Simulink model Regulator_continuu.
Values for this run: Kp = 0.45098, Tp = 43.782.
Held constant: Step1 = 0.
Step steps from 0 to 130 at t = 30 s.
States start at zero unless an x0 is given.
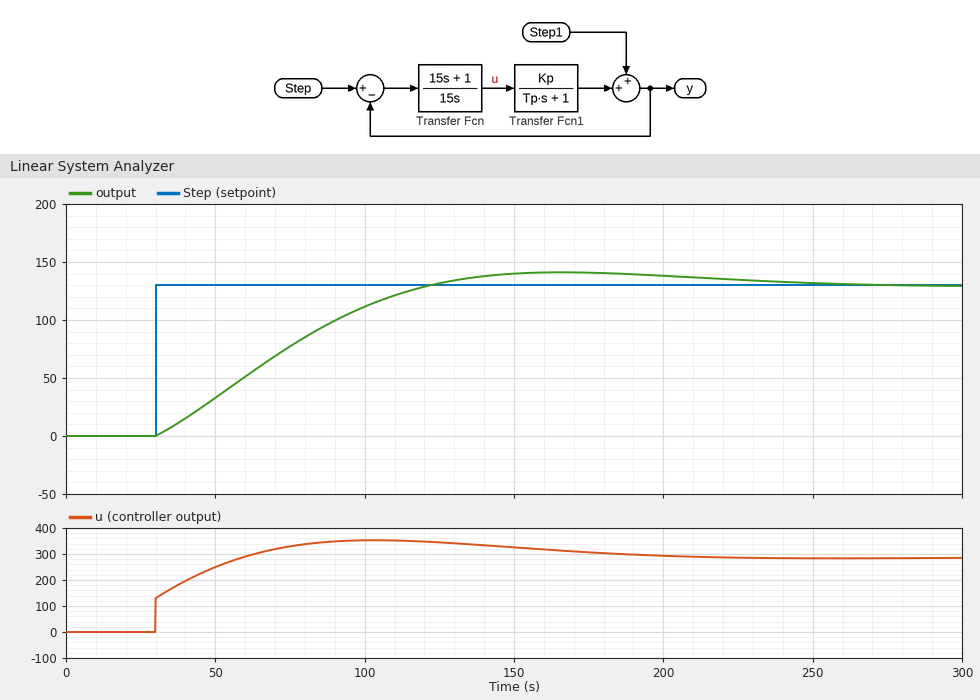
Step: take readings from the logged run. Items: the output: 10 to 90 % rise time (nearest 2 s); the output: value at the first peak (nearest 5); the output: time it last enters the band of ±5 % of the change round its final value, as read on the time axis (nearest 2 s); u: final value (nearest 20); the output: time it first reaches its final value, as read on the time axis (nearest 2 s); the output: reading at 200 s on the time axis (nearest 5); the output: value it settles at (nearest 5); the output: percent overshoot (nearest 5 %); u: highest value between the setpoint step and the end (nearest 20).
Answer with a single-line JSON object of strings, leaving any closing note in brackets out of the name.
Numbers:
{"the output: 10 to 90 % rise time": "66 s", "the output: value at the first peak": "140", "the output: time it last enters the band of ±5 % of the change round its final value, as read on the time axis": "212 s", "u: final value": "280", "the output: time it first reaches its final value, as read on the time axis": "122 s", "the output: reading at 200 s on the time axis": "140", "the output: value it settles at": "130", "the output: percent overshoot": "10 %", "u: highest value between the setpoint step and the end": "360"}
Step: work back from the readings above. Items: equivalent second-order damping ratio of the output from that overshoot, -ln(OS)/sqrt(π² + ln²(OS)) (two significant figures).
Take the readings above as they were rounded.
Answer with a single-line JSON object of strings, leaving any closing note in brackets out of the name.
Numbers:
{"equivalent second-order damping ratio of the output from that overshoot, -ln(OS)/sqrt(π² + ln²(OS))": "0.59"}
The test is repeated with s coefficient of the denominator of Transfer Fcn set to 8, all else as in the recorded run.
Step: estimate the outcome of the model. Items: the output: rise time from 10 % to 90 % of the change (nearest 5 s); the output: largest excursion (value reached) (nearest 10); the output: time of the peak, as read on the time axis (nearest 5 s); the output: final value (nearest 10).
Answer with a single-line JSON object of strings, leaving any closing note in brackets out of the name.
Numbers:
{"the output: rise time from 10 % to 90 % of the change": "40 s", "the output: largest excursion (value reached)": "150", "the output: time of the peak, as read on the time axis": "120 s", "the output: final value": "130"}
